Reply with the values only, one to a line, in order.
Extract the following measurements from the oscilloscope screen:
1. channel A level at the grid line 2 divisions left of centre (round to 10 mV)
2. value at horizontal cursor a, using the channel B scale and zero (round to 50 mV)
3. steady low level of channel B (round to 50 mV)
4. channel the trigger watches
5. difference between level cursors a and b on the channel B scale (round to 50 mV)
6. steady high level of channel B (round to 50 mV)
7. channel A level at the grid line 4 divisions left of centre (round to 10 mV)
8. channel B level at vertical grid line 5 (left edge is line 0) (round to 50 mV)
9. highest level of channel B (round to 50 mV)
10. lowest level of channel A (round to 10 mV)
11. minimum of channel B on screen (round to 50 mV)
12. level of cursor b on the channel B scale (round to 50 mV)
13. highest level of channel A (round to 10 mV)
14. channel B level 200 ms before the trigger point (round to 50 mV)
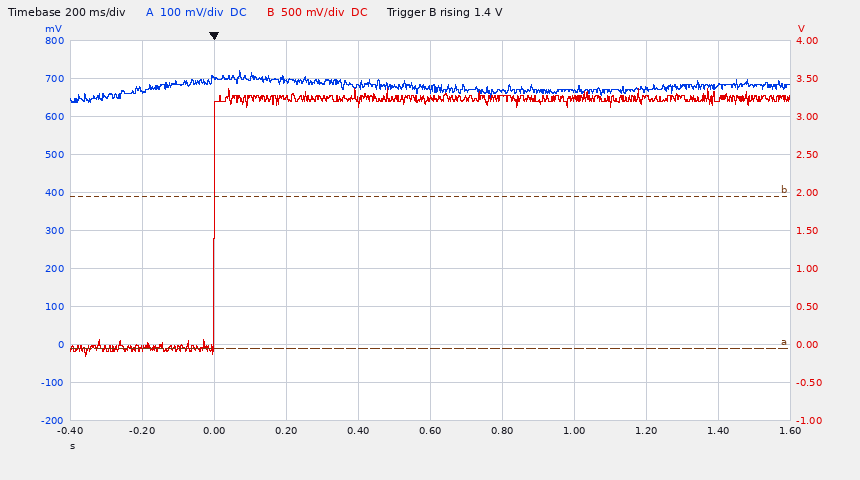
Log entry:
700 mV
-50 mV
-50 mV
channel B
2.00 V
3.25 V
670 mV
3.25 V
3.35 V
640 mV
-150 mV
1.95 V
720 mV
-50 mV
